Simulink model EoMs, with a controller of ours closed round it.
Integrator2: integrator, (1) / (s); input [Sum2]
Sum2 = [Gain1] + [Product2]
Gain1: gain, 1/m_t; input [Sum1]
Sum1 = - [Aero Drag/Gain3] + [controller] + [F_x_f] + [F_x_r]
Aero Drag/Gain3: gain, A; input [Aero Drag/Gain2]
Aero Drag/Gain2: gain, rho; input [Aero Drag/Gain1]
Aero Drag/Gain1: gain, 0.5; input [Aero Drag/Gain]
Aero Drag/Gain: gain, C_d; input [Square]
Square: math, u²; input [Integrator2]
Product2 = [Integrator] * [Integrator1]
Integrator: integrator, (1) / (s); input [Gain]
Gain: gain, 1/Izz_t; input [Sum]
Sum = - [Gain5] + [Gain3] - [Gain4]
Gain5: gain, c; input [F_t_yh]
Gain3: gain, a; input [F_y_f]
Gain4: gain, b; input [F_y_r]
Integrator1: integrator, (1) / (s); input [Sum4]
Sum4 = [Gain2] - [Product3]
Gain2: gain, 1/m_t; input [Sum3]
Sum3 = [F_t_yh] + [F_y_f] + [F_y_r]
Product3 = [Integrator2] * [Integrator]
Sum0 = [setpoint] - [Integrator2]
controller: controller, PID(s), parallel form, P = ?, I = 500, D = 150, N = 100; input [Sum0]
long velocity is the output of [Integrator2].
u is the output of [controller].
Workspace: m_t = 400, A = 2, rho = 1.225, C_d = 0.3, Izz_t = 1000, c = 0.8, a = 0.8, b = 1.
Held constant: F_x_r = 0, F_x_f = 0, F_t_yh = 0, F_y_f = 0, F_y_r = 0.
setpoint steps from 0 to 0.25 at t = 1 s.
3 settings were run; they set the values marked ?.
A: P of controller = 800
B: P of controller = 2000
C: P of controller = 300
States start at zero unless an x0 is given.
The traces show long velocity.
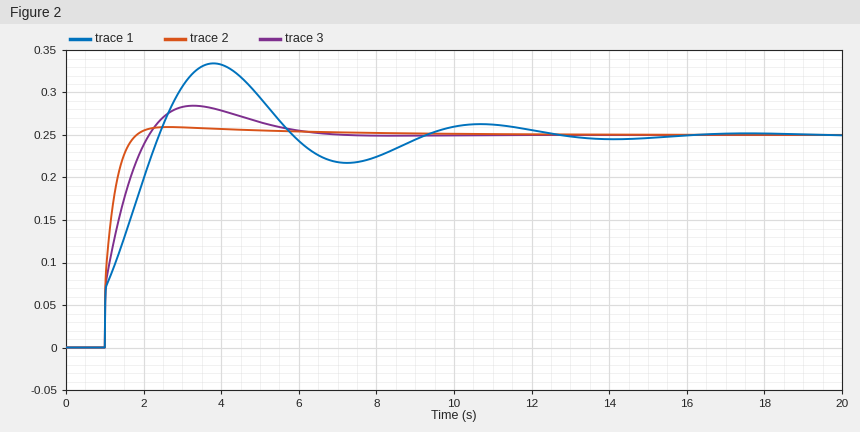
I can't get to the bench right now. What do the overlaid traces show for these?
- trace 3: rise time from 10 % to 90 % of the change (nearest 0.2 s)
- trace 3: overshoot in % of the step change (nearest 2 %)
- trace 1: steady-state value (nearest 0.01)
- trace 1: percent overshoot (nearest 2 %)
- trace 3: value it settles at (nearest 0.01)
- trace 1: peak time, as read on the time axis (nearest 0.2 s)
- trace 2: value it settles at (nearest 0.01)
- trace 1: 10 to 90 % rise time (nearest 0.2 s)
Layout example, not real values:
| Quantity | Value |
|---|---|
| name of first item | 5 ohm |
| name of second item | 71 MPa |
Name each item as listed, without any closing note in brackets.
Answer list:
| Quantity | Value |
|---|---|
| trace 3: rise time from 10 % to 90 % of the change | 0.8 s |
| trace 3: overshoot in % of the step change | 14 % |
| trace 1: steady-state value | 0.25 |
| trace 1: percent overshoot | 34 % |
| trace 3: value it settles at | 0.25 |
| trace 1: peak time, as read on the time axis | 3.8 s |
| trace 2: value it settles at | 0.25 |
| trace 1: 10 to 90 % rise time | 1.2 s |
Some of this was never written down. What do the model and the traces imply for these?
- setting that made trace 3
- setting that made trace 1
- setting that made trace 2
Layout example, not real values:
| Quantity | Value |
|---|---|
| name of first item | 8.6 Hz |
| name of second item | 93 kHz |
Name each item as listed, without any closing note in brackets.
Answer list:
| Quantity | Value |
|---|---|
| setting that made trace 3 | A |
| setting that made trace 1 | C |
| setting that made trace 2 | B |
